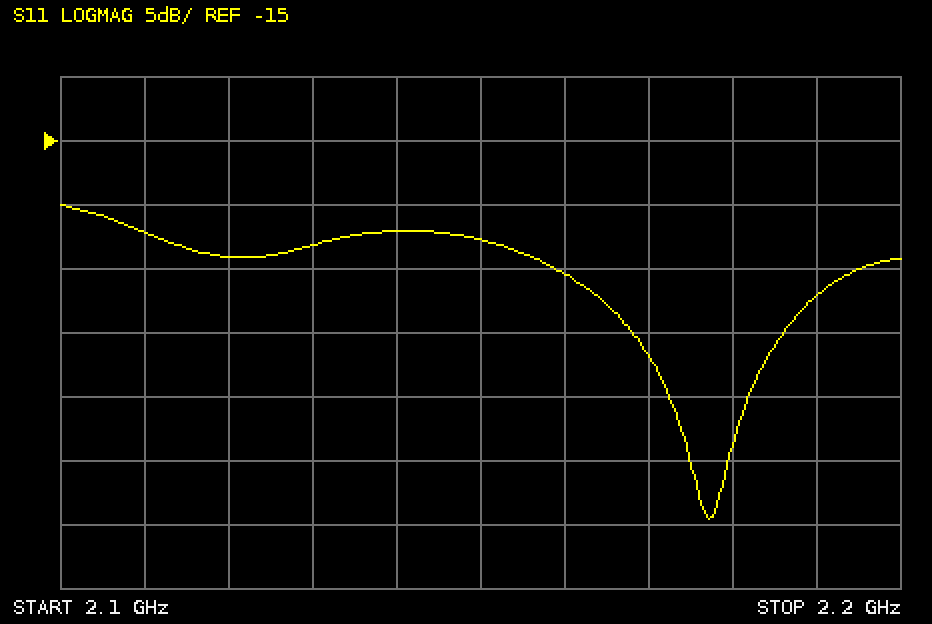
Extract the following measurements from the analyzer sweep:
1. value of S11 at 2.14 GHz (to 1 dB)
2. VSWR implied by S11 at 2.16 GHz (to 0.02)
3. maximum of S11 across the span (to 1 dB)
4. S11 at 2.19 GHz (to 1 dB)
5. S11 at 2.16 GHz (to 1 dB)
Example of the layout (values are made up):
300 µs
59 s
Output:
-22 dB
1.12
-20 dB
-27 dB
-25 dB
